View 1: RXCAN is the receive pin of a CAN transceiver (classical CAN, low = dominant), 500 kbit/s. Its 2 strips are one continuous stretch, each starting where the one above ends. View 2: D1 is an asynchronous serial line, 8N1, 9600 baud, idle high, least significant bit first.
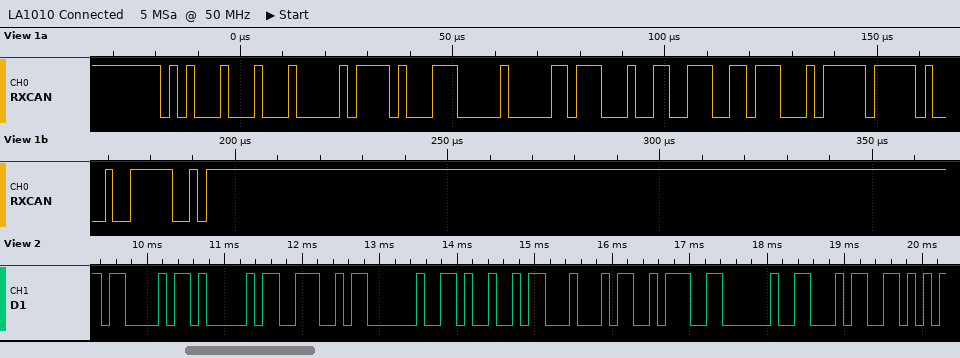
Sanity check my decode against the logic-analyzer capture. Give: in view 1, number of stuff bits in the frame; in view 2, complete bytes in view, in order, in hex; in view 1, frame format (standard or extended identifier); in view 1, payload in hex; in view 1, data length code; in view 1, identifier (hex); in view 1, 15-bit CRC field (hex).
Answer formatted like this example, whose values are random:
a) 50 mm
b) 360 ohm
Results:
a) 6
b) 43 41 4E 20 49 44 3A 20 34
c) standard
d) 1E 8E 00 5C 4C E6 E2 FF
e) 8
f) 0x511
g) 0x713E
